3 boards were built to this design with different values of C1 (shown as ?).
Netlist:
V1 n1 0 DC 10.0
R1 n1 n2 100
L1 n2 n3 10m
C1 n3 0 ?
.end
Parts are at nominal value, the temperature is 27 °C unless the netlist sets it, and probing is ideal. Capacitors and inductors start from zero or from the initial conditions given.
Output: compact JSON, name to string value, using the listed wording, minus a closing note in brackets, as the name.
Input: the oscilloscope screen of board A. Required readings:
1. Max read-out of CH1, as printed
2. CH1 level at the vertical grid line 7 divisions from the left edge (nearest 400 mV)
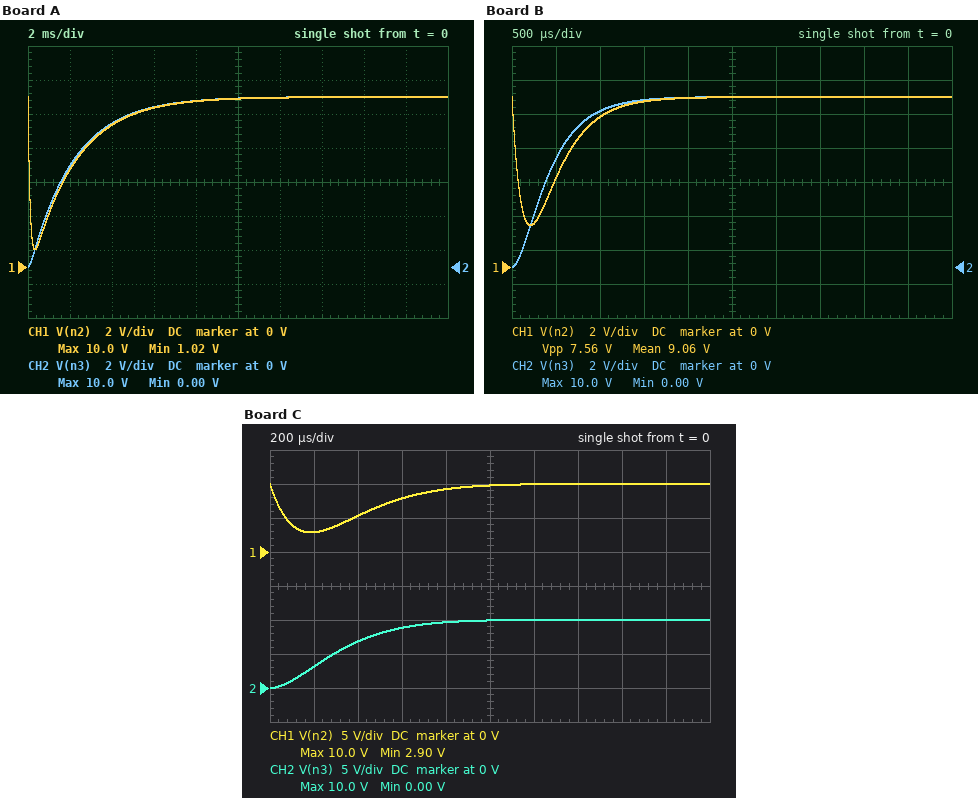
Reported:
{"Max read-out of CH1, as printed": "10.0 V", "CH1 level at the vertical grid line 7 divisions from the left edge": "10.0 V"}
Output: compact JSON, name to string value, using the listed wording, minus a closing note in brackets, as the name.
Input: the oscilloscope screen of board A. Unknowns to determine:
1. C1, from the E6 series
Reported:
{"C1, from the E6 series": "22 µF"}
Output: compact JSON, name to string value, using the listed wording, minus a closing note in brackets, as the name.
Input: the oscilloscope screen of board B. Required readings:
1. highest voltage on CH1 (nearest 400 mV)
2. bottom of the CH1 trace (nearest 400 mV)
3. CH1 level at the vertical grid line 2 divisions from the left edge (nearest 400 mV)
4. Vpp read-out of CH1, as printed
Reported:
{"highest voltage on CH1": "10.0 V", "bottom of the CH1 trace": "2.4 V", "CH1 level at the vertical grid line 2 divisions from the left edge": "8.8 V", "Vpp read-out of CH1, as printed": "7.56 V"}
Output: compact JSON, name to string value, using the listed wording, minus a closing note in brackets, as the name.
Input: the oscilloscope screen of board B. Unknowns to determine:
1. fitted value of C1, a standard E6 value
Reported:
{"fitted value of C1, a standard E6 value": "4.7 µF"}
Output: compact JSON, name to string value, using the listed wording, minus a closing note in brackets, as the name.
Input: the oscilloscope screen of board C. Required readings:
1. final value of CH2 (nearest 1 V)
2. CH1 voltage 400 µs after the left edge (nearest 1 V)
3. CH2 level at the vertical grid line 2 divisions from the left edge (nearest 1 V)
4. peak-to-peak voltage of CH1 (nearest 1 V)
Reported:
{"final value of CH2": "10 V", "CH1 voltage 400 µs after the left edge": "5 V", "CH2 level at the vertical grid line 2 divisions from the left edge": "7 V", "peak-to-peak voltage of CH1": "7 V"}
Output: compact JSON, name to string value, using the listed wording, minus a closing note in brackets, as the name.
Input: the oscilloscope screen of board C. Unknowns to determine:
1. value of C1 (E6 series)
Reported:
{"value of C1": "3.3 µF"}
